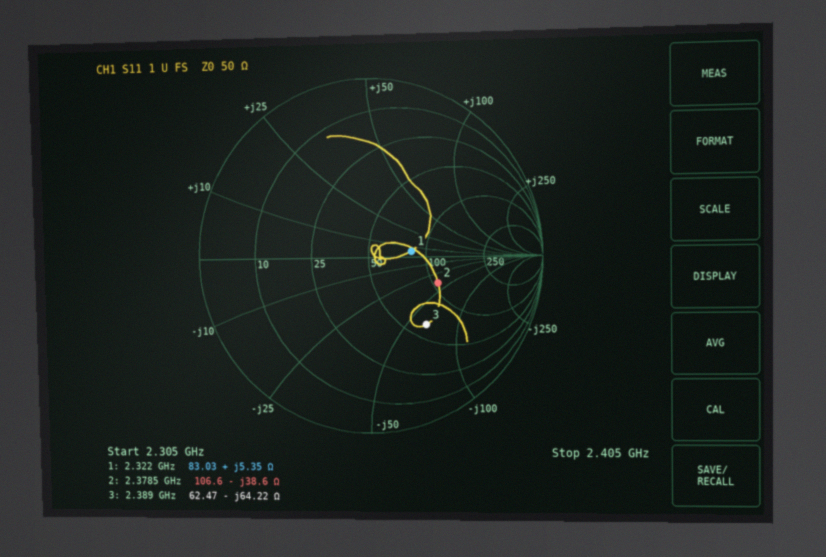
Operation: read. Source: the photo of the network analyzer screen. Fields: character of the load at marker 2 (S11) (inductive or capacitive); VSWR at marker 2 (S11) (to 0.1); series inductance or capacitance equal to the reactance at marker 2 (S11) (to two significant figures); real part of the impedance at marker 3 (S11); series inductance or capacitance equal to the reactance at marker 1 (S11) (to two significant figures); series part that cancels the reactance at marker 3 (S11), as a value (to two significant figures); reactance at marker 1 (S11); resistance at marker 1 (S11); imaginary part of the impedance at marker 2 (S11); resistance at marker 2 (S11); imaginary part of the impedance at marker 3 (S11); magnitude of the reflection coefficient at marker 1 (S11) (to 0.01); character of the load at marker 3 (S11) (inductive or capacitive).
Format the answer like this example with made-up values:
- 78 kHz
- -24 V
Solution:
- capacitive
- 2.5
- 1.7 pF
- 62.47 Ω
- 370 pH
- 4.3 nH
- +5.35 Ω
- 83.03 Ω
- -38.6 Ω
- 106.6 Ω
- -64.22 Ω
- 0.25
- capacitive
